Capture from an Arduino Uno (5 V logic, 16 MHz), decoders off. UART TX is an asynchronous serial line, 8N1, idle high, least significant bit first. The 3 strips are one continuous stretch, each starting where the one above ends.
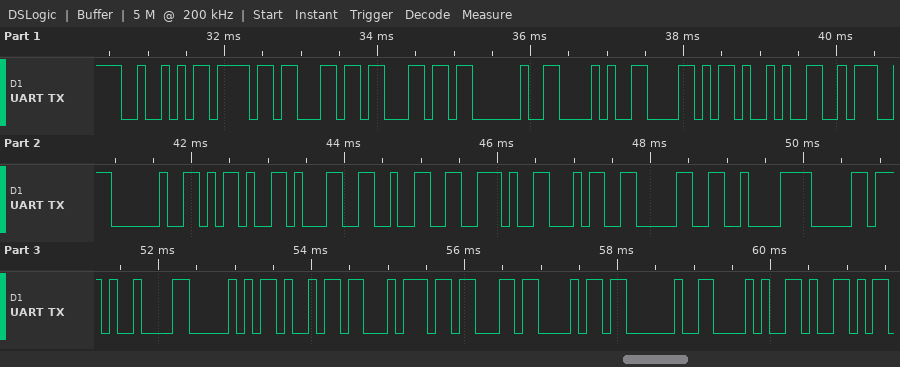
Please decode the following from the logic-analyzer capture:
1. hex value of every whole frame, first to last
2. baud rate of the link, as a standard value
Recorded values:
0x52 0x6F 0x6C 0x6C 0x20 0x28 0x58 0x29 0x3A 0x20 0x2D 0x31 0x32 0x2E 0x34 0x30 0xC2 0xB0 0x09 0x50 0x69 0x74 0x63 0x68 0x20 0x28 0x59
9600 baud
